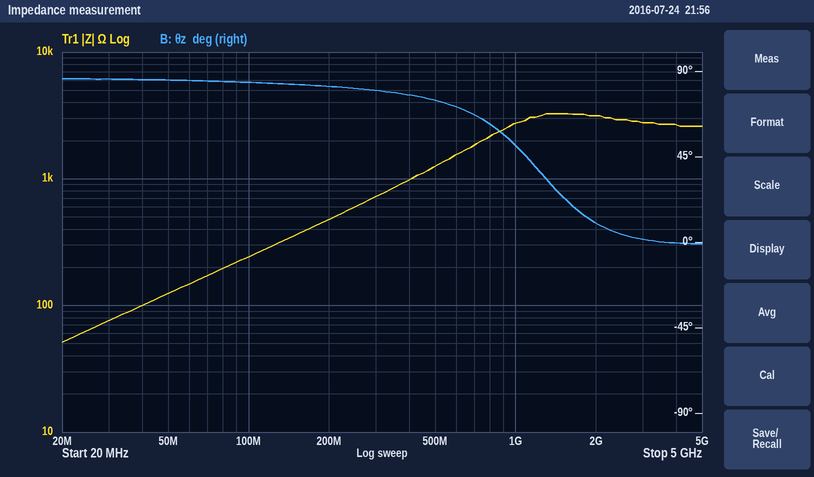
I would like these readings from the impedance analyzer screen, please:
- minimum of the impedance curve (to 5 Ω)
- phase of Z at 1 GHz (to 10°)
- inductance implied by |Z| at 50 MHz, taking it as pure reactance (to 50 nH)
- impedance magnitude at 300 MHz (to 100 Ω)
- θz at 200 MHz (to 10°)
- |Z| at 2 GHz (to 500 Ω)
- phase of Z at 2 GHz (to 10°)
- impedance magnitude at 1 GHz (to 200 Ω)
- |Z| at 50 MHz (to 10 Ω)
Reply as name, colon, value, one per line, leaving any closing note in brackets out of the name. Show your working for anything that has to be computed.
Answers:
minimum of the impedance curve: 50 Ω
phase of Z at 1 GHz: 50°
inductance implied by |Z| at 50 MHz, taking it as pure reactance: L = 120 Ω/(2π × 50 MHz) ≈ 382 nH, so 400 nH to the nearest 50 nH
impedance magnitude at 300 MHz: 700 Ω
θz at 200 MHz: 80°
|Z| at 2 GHz: 3.0 kΩ
phase of Z at 2 GHz: 10°
impedance magnitude at 1 GHz: 2.8 kΩ
|Z| at 50 MHz: 120 Ω
